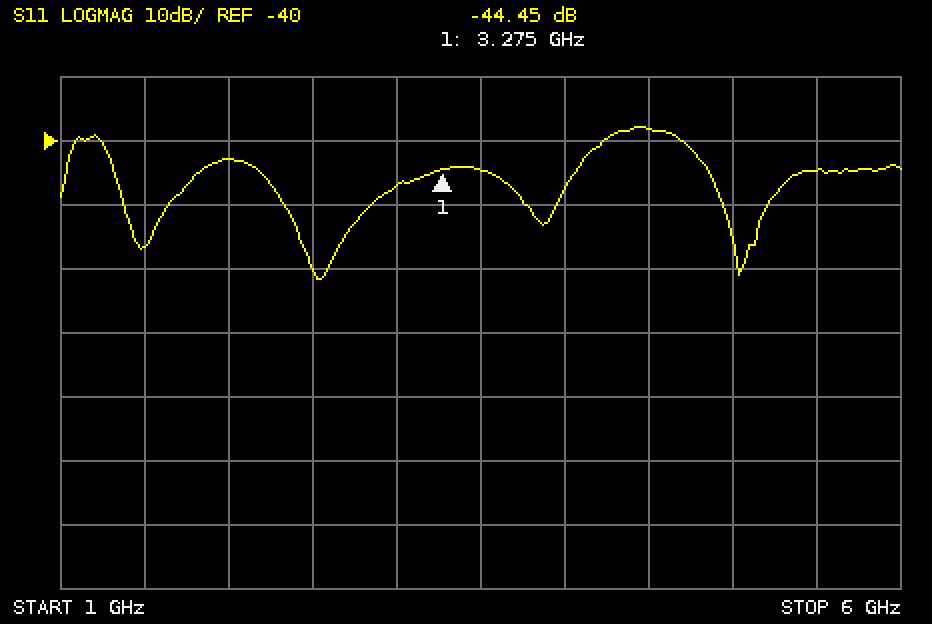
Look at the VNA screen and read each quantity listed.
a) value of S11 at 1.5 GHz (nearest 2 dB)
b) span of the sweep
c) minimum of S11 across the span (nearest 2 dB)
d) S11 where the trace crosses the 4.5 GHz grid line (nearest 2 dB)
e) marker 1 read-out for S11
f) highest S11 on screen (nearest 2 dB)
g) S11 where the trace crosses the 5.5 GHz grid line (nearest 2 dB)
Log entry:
-56 dB
5 GHz
-62 dB
-38 dB
-44.45 dB
-38 dB
-44 dB
